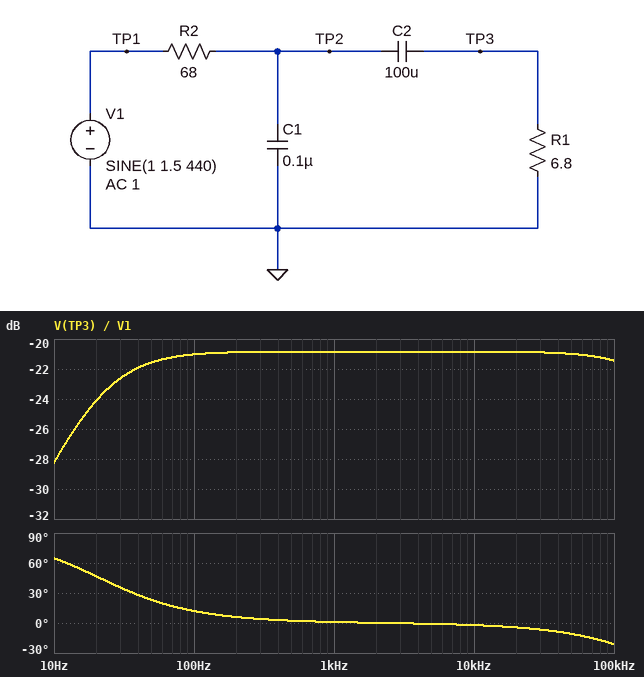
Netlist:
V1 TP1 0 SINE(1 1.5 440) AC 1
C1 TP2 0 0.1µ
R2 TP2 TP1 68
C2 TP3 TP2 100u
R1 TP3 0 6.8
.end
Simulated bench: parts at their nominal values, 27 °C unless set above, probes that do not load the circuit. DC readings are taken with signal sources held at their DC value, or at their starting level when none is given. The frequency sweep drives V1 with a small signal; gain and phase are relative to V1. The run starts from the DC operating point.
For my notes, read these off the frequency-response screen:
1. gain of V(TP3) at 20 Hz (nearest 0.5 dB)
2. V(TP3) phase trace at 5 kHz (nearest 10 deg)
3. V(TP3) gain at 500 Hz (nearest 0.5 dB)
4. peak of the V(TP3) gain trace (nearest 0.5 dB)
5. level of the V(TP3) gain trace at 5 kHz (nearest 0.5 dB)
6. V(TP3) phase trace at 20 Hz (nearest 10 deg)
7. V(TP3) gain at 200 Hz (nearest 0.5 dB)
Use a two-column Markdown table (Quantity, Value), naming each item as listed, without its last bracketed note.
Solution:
| Quantity | Value |
|---|---|
| gain of V(TP3) at 20 Hz | -24.0 dB |
| V(TP3) phase trace at 5 kHz | 0 deg |
| V(TP3) gain at 500 Hz | -21.0 dB |
| peak of the V(TP3) gain trace | -21.0 dB |
| level of the V(TP3) gain trace at 5 kHz | -21.0 dB |
| V(TP3) phase trace at 20 Hz | 50 deg |
| V(TP3) gain at 200 Hz | -21.0 dB |
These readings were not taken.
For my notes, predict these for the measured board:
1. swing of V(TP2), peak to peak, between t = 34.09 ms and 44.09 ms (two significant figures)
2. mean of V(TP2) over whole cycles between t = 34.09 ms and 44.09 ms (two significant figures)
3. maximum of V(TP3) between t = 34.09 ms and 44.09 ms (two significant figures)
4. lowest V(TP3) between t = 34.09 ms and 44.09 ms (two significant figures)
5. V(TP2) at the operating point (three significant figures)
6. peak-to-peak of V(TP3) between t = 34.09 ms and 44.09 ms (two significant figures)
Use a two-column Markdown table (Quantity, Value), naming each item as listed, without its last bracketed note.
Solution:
| Quantity | Value |
|---|---|
| swing of V(TP2), peak to peak, between t = 34.09 ms and 44.09 ms | 310 mV |
| mean of V(TP2) over whole cycles between t = 34.09 ms and 44.09 ms | 1.0 V |
| maximum of V(TP3) between t = 34.09 ms and 44.09 ms | 140 mV |
| lowest V(TP3) between t = 34.09 ms and 44.09 ms | -140 mV |
| V(TP2) at the operating point | 1.00 V |
| peak-to-peak of V(TP3) between t = 34.09 ms and 44.09 ms | 270 mV |
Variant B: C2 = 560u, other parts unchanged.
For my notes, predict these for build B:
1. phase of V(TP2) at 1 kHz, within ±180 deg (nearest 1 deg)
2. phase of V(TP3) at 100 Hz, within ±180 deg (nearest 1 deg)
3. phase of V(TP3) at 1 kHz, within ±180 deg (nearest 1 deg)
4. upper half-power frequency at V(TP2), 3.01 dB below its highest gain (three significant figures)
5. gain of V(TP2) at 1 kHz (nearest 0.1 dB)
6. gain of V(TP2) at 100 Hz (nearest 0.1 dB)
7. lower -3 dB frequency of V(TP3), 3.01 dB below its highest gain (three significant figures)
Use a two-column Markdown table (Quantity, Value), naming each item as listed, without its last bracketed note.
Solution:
| Quantity | Value |
|---|---|
| phase of V(TP2) at 1 kHz, within ±180 deg | -2 deg |
| phase of V(TP3) at 100 Hz, within ±180 deg | 2 deg |
| phase of V(TP3) at 1 kHz, within ±180 deg | 0 deg |
| upper half-power frequency at V(TP2), 3.01 dB below its highest gain | 3.83 Hz |
| gain of V(TP2) at 1 kHz | -20.8 dB |
| gain of V(TP2) at 100 Hz | -20.1 dB |
| lower -3 dB frequency of V(TP3), 3.01 dB below its highest gain | 3.80 Hz |
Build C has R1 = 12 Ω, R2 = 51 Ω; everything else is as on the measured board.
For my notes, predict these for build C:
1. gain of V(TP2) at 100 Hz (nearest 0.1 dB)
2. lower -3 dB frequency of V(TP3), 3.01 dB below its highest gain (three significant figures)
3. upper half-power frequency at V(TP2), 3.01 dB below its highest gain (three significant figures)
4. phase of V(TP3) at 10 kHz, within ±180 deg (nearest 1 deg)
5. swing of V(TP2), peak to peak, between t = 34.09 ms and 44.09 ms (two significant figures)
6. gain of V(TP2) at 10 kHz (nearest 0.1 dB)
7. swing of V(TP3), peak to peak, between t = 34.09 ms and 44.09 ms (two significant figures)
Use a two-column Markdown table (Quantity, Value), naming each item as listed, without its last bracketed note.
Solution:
| Quantity | Value |
|---|---|
| gain of V(TP2) at 100 Hz | -10.3 dB |
| lower -3 dB frequency of V(TP3), 3.01 dB below its highest gain | 25.2 Hz |
| upper half-power frequency at V(TP2), 3.01 dB below its highest gain | 26.2 Hz |
| phase of V(TP3) at 10 kHz, within ±180 deg | -3 deg |
| swing of V(TP2), peak to peak, between t = 34.09 ms and 44.09 ms | 600 mV |
| gain of V(TP2) at 10 kHz | -14.4 dB |
| swing of V(TP3), peak to peak, between t = 34.09 ms and 44.09 ms | 570 mV |
